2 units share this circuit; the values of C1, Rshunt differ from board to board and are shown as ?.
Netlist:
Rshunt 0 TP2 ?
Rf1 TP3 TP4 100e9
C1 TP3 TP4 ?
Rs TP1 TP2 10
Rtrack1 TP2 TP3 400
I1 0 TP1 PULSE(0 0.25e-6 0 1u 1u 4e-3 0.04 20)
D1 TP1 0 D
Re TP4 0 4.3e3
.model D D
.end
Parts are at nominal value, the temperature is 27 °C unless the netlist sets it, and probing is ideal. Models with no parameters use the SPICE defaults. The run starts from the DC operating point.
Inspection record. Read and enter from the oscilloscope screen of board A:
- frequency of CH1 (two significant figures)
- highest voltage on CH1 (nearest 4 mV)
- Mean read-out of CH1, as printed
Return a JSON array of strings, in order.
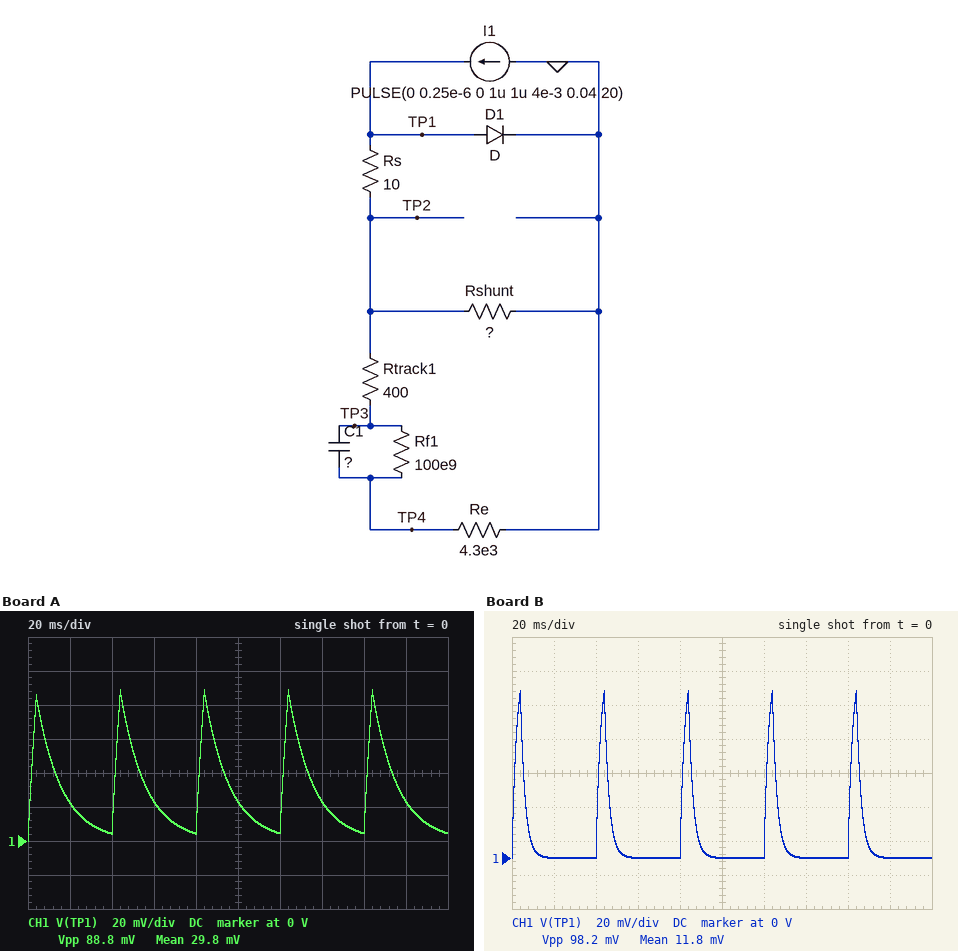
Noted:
["25 Hz", "88 mV", "29.8 mV"]
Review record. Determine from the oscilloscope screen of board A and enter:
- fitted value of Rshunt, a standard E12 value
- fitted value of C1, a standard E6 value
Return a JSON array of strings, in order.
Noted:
["1.2 MΩ", "10 nF"]
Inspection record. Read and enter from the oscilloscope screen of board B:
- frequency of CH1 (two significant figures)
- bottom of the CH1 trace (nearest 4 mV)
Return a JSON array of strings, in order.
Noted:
["25 Hz", "0 V"]
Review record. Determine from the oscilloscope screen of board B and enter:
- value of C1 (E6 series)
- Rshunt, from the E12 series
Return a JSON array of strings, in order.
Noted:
["4.7 nF", "470 kΩ"]
